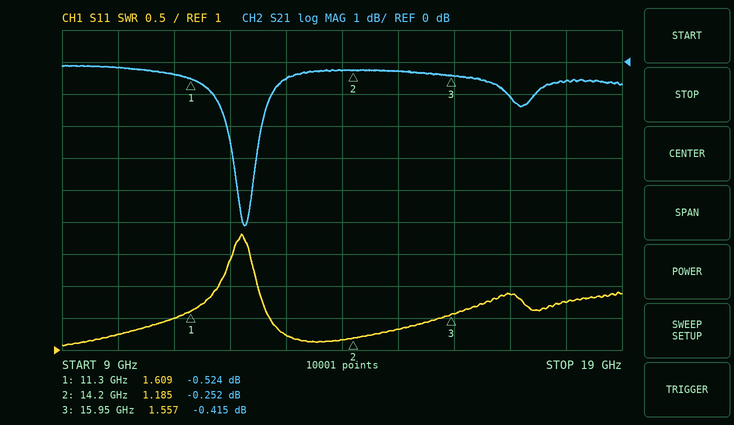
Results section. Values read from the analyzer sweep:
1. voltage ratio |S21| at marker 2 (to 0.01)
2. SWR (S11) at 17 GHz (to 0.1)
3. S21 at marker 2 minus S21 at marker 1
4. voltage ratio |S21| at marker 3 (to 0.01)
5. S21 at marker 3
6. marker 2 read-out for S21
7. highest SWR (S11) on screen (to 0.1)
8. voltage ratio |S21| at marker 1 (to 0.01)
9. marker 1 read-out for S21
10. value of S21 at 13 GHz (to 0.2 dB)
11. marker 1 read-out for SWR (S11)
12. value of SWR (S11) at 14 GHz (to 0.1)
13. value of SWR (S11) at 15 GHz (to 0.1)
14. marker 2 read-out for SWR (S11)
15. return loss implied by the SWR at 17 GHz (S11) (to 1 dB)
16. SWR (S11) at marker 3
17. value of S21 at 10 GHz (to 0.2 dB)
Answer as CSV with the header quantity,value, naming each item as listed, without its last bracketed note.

quantity,value
voltage ratio |S21| at marker 2,0.97
SWR (S11) at 17 GHz,1.9
S21 at marker 2 minus S21 at marker 1,0.272 dB
voltage ratio |S21| at marker 3,0.95
S21 at marker 3,-0.415 dB
marker 2 read-out for S21,-0.252 dB
highest SWR (S11) on screen,2.8
voltage ratio |S21| at marker 1,0.94
marker 1 read-out for S21,-0.524 dB
value of S21 at 13 GHz,-0.6 dB
marker 1 read-out for SWR,1.609
value of SWR (S11) at 14 GHz,1.2
value of SWR (S11) at 15 GHz,1.3
marker 2 read-out for SWR,1.185
return loss implied by the SWR at 17 GHz (S11),10 dB
SWR (S11) at marker 3,1.557
value of S21 at 10 GHz,-0.2 dB
